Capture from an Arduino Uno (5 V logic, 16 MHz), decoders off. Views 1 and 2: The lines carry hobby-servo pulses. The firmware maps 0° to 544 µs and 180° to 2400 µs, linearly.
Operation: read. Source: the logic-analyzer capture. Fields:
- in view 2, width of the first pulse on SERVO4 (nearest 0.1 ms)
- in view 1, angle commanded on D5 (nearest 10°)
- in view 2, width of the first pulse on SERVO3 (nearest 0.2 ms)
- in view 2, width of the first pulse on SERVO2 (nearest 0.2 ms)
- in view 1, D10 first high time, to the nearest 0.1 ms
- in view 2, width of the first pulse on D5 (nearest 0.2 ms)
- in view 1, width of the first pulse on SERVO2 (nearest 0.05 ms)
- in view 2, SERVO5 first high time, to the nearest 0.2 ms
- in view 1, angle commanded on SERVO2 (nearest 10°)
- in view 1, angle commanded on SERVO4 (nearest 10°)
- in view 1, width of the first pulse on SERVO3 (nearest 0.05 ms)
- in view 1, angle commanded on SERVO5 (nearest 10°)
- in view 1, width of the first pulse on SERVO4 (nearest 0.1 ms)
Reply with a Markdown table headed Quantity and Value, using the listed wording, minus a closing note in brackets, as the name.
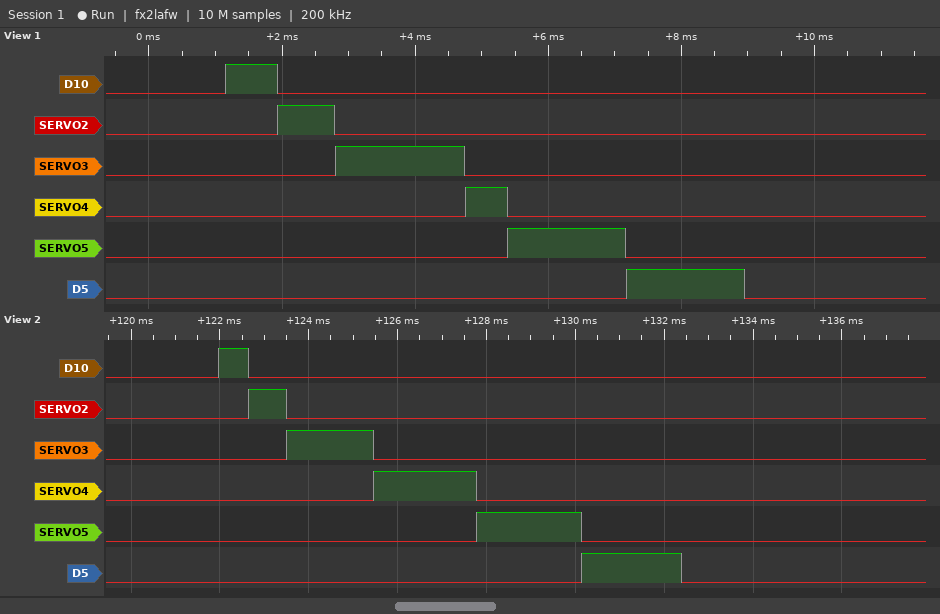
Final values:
| Quantity | Value |
|---|---|
| in view 2, width of the first pulse on SERVO4 | 2.3 ms |
| in view 1, angle commanded on D5 | 120° |
| in view 2, width of the first pulse on SERVO3 | 2.0 ms |
| in view 2, width of the first pulse on SERVO2 | 0.8 ms |
| in view 1, D10 first high time, to the nearest 0.1 ms | 0.8 ms |
| in view 2, width of the first pulse on D5 | 2.2 ms |
| in view 1, width of the first pulse on SERVO2 | 0.85 ms |
| in view 2, SERVO5 first high time, to the nearest 0.2 ms | 2.4 ms |
| in view 1, angle commanded on SERVO2 | 30° |
| in view 1, angle commanded on SERVO4 | 10° |
| in view 1, width of the first pulse on SERVO3 | 1.95 ms |
| in view 1, angle commanded on SERVO5 | 120° |
| in view 1, width of the first pulse on SERVO4 | 0.6 ms |
